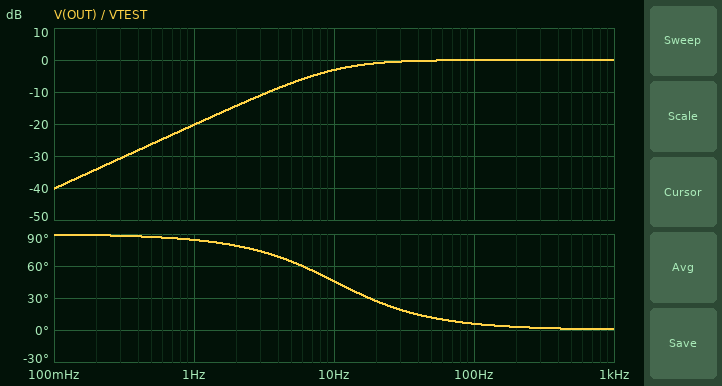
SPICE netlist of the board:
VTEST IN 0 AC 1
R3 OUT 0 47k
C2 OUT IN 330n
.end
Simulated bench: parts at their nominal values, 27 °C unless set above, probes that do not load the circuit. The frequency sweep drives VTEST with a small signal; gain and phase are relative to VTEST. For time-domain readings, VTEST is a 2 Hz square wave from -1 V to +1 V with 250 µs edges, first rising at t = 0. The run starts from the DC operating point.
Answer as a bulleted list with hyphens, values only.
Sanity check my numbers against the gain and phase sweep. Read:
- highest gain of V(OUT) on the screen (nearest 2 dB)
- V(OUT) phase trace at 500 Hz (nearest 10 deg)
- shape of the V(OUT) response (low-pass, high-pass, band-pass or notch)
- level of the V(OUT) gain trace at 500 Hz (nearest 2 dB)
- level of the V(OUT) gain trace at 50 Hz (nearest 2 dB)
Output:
- 0 dB
- 0 deg
- high-pass
- 0 dB
- 0 dB
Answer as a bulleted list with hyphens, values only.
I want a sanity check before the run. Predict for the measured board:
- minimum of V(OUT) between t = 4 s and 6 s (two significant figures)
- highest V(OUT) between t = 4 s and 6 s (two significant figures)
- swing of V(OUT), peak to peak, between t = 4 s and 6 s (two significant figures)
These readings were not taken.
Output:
- -2.0 V
- 2.0 V
- 4.0 V
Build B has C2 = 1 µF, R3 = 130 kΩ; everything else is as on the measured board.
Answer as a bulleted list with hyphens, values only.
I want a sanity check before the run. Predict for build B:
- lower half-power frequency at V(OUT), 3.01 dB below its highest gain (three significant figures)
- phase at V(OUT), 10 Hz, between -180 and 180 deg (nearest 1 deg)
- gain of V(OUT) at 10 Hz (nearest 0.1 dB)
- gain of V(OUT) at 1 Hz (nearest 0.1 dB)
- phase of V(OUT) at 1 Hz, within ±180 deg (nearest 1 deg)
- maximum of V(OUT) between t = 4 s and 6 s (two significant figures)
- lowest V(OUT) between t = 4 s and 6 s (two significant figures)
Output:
- 1.22 Hz
- 7 deg
- -0.1 dB
- -4.0 dB
- 51 deg
- 1.7 V
- -1.7 V
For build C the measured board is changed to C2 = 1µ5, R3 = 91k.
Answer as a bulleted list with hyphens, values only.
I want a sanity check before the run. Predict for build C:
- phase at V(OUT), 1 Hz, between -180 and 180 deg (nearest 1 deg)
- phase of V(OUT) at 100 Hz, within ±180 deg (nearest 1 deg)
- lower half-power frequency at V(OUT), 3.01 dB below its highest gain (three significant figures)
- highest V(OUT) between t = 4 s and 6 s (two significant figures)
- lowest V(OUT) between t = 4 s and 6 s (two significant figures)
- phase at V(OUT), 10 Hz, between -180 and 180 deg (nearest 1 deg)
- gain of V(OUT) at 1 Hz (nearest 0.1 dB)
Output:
- 49 deg
- 1 deg
- 1.17 Hz
- 1.7 V
- -1.7 V
- 7 deg
- -3.7 dB
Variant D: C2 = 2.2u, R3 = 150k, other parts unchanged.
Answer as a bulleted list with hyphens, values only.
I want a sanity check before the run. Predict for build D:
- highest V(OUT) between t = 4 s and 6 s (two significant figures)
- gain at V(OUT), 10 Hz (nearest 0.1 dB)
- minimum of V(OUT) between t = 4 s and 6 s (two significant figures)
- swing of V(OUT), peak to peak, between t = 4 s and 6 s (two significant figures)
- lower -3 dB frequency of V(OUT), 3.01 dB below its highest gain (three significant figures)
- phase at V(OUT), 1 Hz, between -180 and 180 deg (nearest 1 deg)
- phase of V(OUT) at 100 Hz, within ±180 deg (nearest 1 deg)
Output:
- 1.4 V
- 0 dB
- -1.4 V
- 2.7 V
- 482 mHz
- 26 deg
- 0 deg
